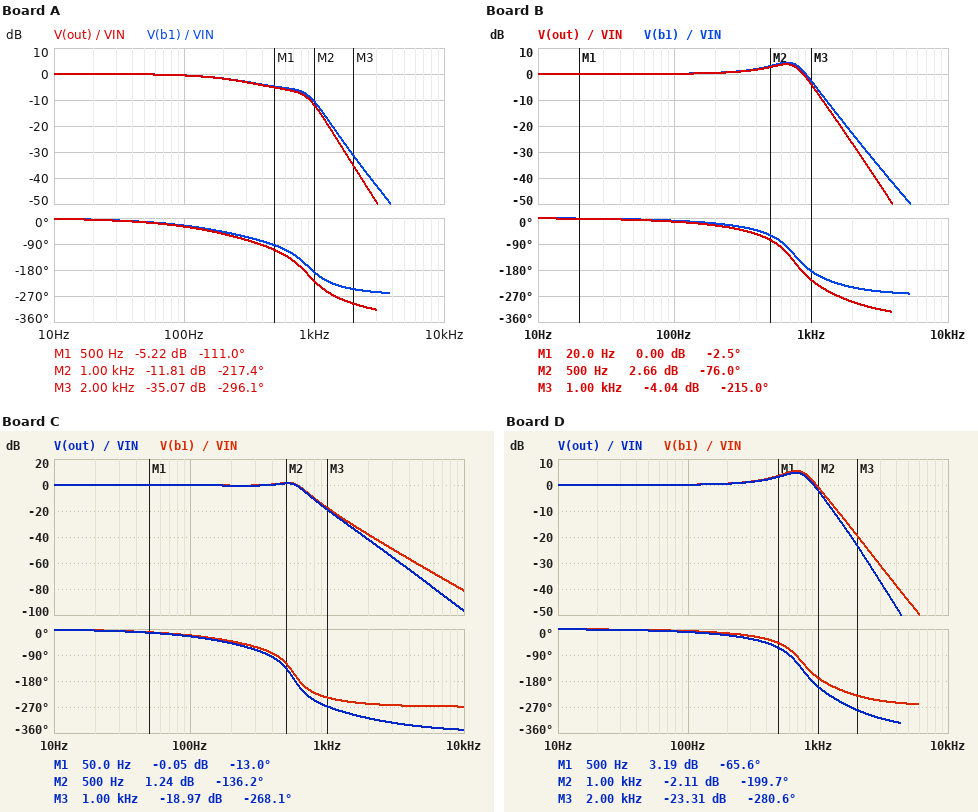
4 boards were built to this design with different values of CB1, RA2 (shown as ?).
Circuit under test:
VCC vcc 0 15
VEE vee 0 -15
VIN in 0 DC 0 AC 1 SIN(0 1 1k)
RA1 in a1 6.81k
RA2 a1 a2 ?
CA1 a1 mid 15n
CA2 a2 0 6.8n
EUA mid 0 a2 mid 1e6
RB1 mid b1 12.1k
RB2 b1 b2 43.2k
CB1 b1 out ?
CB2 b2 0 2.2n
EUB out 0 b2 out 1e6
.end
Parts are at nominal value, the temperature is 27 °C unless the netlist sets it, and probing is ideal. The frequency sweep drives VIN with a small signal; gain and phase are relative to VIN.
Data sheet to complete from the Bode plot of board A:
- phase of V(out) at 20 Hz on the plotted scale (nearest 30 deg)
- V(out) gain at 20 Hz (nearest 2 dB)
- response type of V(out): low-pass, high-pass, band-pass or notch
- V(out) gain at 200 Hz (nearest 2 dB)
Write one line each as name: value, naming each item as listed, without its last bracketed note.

phase of V(out) at 20 Hz on the plotted scale: 0 deg
V(out) gain at 20 Hz: 0 dB
response type of V(out): low-pass, high-pass, band-pass or notch: low-pass
V(out) gain at 200 Hz: -2 dB
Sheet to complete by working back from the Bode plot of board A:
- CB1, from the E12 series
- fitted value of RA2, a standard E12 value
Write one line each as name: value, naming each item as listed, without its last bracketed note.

CB1, from the E12 series: 27 nF
fitted value of RA2, a standard E12 value: 100 kΩ
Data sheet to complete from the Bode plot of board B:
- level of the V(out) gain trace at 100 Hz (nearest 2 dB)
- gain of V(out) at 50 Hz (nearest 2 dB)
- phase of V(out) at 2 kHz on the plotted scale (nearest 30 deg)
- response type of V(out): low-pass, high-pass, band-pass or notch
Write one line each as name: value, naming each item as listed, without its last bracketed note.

level of the V(out) gain trace at 100 Hz: 0 dB
gain of V(out) at 50 Hz: 0 dB
phase of V(out) at 2 kHz on the plotted scale: -300 deg
response type of V(out): low-pass, high-pass, band-pass or notch: low-pass
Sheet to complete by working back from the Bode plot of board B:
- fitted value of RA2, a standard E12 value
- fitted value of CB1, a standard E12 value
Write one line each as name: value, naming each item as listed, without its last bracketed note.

fitted value of RA2, a standard E12 value: 27 kΩ
fitted value of CB1, a standard E12 value: 39 nF
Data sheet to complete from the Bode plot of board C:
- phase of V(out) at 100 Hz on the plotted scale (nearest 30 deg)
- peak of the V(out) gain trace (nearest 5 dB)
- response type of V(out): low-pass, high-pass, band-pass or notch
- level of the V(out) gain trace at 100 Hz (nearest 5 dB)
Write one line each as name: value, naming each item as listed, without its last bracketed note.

phase of V(out) at 100 Hz on the plotted scale: -30 deg
peak of the V(out) gain trace: 0 dB
response type of V(out): low-pass, high-pass, band-pass or notch: low-pass
level of the V(out) gain trace at 100 Hz: 0 dB
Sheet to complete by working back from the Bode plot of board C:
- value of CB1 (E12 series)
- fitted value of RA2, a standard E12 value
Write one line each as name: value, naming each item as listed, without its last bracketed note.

value of CB1: 68 nF
fitted value of RA2, a standard E12 value: 82 kΩ
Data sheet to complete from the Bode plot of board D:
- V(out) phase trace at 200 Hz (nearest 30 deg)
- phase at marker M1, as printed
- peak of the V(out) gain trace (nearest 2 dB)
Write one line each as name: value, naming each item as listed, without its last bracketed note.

V(out) phase trace at 200 Hz: -30 deg
phase at marker M1, as printed: -65.6 deg
peak of the V(out) gain trace: 4 dB
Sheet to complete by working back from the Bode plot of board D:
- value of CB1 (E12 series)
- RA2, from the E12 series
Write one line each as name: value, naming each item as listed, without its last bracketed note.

value of CB1: 39 nF
RA2, from the E12 series: 18 kΩ
